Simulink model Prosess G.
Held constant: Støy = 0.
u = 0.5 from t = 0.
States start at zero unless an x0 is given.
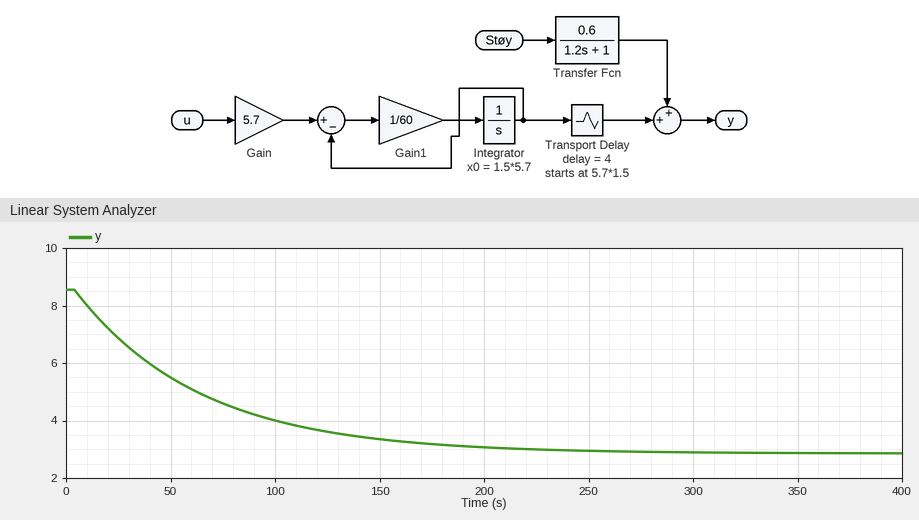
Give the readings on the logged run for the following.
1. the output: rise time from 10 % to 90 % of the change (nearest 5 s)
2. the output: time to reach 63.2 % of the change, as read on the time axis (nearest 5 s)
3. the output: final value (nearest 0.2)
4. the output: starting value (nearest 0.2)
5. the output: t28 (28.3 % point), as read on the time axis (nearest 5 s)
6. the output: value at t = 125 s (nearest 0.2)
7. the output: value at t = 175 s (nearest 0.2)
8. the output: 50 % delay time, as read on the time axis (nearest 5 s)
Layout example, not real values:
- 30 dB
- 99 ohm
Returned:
- 130 s
- 65 s
- 2.8
- 8.6
- 25 s
- 3.6
- 3.2
- 45 s
